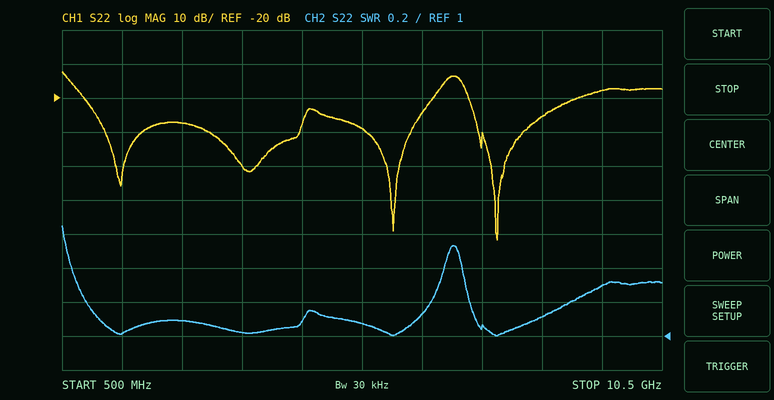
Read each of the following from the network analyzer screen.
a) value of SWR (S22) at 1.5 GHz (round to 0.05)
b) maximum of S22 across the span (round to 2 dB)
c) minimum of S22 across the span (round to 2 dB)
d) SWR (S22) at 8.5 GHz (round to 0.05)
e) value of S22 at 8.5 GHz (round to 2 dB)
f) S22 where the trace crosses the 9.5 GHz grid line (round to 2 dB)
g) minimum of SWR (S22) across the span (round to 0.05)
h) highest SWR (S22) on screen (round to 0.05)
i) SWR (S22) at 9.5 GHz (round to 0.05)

1.00
-12 dB
-62 dB
1.10
-26 dB
-18 dB
1.00
1.65
1.30
